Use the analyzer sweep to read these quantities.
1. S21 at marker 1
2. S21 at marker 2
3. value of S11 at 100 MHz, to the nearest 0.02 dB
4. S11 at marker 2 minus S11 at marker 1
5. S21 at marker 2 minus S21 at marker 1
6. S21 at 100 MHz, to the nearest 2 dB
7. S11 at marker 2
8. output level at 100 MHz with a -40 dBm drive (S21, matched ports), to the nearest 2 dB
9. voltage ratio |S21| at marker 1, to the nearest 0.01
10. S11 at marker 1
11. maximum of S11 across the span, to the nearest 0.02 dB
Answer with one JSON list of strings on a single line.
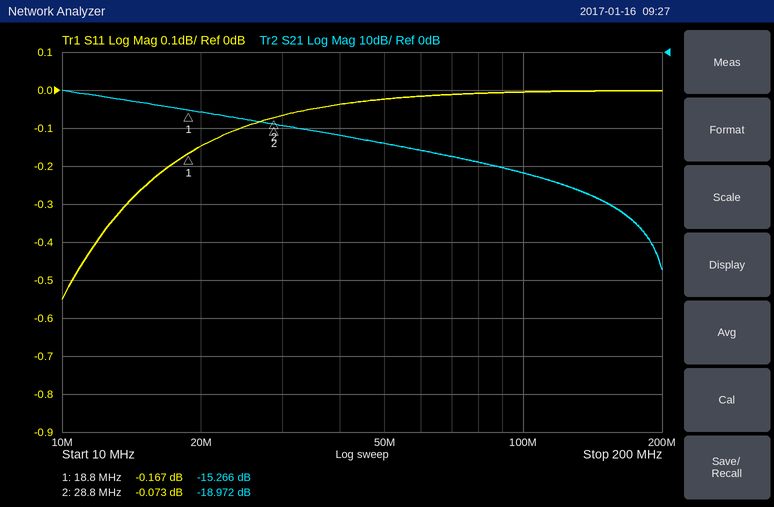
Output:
["-15.266 dB", "-18.972 dB", "0.00 dB", "0.094 dB", "-3.706 dB", "-32 dB", "-0.073 dB", "-72 dBm", "0.17", "-0.167 dB", "0.00 dB"]
